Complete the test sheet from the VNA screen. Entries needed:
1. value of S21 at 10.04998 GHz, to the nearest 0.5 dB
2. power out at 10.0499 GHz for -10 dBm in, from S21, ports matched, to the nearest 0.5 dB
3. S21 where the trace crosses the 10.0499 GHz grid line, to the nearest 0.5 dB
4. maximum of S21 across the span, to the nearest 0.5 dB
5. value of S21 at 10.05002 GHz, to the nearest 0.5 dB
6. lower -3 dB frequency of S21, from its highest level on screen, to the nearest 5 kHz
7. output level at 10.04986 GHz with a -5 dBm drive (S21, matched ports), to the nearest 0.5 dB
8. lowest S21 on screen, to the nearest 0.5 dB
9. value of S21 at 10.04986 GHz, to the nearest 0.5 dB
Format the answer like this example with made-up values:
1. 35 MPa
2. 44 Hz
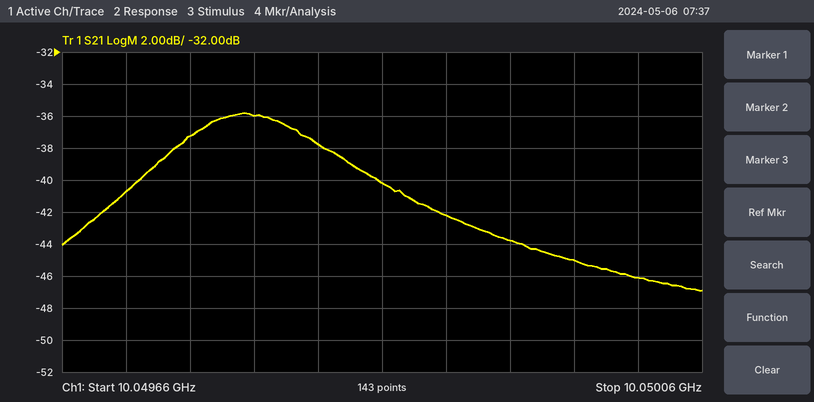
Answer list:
1. -45.0 dB
2. -52.0 dBm
3. -42.0 dB
4. -36.0 dB
5. -46.0 dB
6. 10.049720 GHz
7. -45.0 dBm
8. -47.0 dB
9. -40.0 dB
